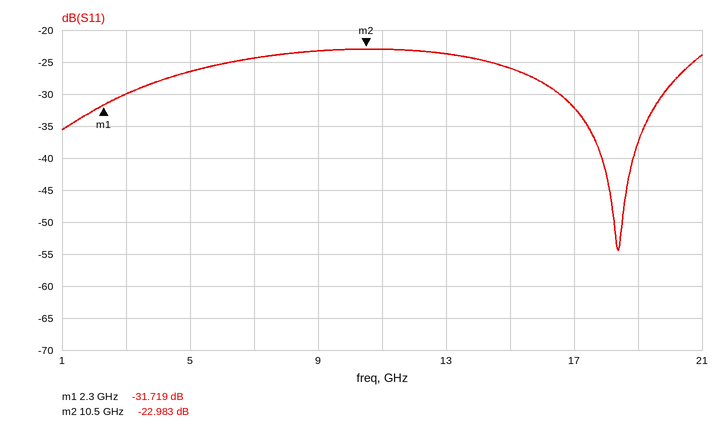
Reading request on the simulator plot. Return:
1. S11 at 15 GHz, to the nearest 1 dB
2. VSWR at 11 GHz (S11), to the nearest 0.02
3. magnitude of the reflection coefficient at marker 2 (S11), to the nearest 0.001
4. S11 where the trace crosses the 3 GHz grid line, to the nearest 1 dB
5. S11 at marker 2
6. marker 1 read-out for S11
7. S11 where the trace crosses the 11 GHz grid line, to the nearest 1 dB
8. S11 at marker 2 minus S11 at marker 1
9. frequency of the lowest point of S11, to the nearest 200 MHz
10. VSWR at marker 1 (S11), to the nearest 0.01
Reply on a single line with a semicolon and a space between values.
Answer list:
-26 dB; 1.16; 0.071; -30 dB; -22.983 dB; -31.719 dB; -23 dB; 8.736 dB; 18.4 GHz; 1.05
